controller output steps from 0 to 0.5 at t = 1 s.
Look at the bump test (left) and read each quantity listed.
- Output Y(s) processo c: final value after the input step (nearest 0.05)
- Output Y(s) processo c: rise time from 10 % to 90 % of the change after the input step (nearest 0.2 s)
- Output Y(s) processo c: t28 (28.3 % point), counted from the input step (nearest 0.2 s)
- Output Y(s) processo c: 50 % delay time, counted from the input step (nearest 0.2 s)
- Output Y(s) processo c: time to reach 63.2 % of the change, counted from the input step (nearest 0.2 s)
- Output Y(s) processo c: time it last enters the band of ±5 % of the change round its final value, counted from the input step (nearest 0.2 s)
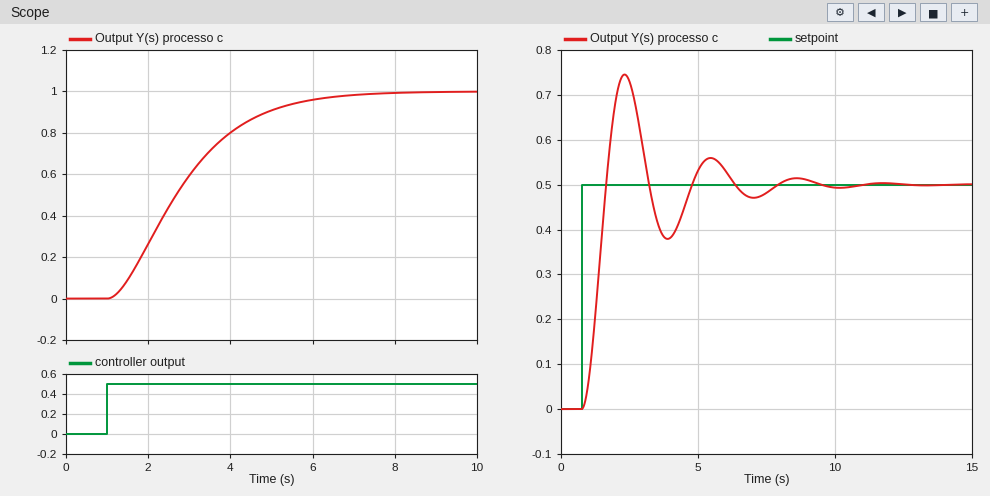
1.00
3.4 s
1.0 s
1.6 s
2.2 s
4.8 s
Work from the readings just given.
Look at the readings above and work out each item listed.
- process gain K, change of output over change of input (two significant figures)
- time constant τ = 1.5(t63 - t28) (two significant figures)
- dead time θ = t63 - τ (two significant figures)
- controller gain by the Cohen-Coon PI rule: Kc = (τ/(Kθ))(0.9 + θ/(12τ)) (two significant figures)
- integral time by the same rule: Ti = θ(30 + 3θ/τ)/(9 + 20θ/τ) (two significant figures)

2.0
1.8 s
0.40 s
2.1
0.91 s
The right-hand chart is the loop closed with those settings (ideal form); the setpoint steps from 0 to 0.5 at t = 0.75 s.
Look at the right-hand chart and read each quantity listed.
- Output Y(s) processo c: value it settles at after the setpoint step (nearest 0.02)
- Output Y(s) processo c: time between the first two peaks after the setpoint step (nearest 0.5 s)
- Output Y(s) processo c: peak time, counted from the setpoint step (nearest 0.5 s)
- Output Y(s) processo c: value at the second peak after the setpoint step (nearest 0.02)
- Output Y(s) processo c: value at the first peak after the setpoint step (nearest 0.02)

0.50
3.0 s
1.5 s
0.56
0.74
